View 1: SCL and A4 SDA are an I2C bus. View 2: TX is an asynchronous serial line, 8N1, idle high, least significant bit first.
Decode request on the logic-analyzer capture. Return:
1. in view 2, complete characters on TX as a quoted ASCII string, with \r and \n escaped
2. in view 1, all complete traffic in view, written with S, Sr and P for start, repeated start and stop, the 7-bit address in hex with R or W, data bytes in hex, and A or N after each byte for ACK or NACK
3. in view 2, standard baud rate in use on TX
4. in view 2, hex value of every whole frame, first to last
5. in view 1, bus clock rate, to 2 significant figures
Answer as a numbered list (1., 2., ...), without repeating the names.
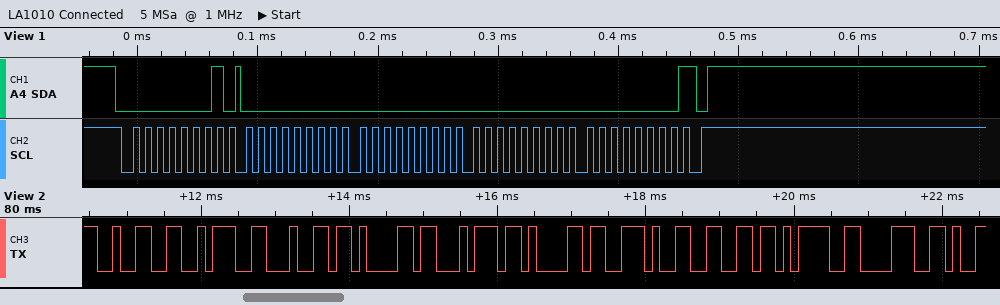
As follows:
1. "2:data.f=8"
2. S 00R A 00 A 00 A 00 A 00 N P
3. 9600 baud
4. 32 3A 64 61 74 61 2E 66 3D 38
5. 100 kHz
